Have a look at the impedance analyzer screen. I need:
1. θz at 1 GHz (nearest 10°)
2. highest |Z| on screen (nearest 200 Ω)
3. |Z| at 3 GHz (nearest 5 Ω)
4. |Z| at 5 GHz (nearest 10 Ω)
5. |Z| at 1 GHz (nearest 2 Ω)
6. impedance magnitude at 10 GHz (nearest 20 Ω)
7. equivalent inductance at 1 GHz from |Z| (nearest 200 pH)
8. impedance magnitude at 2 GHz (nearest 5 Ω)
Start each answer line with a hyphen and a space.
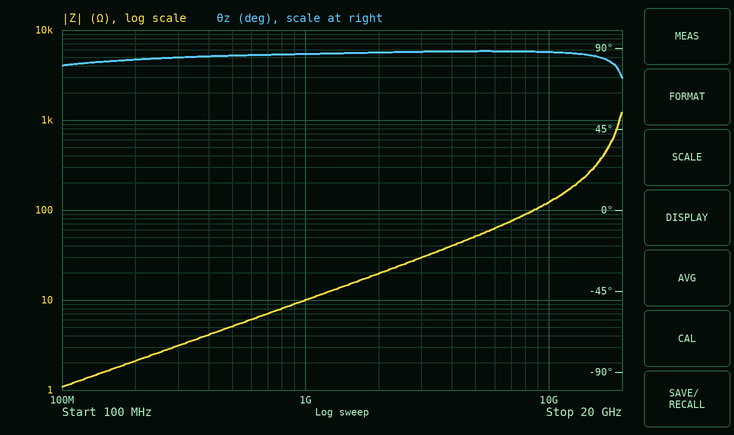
- 90°
- 1.2 kΩ
- 30 Ω
- 50 Ω
- 10 Ω
- 120 Ω
- 1.6 nH
- 20 Ω
